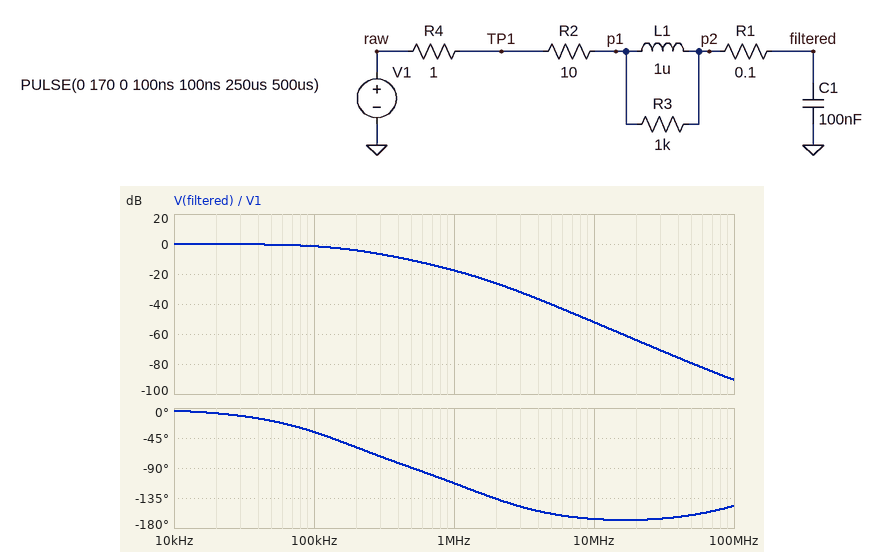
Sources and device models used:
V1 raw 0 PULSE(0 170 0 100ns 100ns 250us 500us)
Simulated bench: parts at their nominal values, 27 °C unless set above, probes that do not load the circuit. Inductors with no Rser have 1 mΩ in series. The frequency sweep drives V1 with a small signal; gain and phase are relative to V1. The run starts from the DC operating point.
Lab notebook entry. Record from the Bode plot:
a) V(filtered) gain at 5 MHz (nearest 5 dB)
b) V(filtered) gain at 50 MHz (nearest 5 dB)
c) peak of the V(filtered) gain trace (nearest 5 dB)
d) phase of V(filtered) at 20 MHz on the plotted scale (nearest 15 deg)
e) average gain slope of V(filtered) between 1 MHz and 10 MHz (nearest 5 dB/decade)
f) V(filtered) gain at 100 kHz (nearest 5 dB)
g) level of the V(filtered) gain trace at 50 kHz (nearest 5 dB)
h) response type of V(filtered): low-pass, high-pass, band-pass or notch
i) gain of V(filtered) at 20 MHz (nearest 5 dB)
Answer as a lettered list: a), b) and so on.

a) -40 dB
b) -80 dB
c) 0 dB
d) -165 deg
e) -35 dB/decade
f) 0 dB
g) 0 dB
h) low-pass
i) -65 dB
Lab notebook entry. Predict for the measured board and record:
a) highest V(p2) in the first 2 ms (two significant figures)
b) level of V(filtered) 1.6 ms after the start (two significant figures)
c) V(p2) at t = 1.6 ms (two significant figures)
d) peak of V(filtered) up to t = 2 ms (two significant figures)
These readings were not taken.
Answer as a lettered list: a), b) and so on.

a) 170 V
b) 170 V
c) 170 V
d) 170 V
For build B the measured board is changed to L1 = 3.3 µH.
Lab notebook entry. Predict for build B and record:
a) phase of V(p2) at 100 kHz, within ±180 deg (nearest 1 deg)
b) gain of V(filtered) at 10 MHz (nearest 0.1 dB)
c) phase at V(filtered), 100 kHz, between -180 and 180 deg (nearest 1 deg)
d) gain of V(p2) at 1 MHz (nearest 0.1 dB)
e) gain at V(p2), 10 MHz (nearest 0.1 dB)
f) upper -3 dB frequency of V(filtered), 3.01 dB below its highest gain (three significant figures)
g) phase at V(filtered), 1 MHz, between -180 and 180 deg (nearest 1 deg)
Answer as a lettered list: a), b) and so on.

a) -38 deg
b) -62.2 dB
c) -39 deg
d) -22.9 dB
e) -60.8 dB
f) 187 kHz
g) -149 deg
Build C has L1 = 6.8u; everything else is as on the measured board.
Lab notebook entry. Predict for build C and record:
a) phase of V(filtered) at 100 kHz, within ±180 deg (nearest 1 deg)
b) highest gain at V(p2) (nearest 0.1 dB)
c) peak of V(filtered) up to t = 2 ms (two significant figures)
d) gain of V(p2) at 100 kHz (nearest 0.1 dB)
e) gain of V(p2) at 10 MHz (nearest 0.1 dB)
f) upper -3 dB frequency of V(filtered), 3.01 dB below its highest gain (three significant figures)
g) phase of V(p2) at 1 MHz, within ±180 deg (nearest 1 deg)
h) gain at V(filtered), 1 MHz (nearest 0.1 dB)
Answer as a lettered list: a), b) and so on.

a) -44 deg
b) 0 dB
c) 180 V
d) -0.1 dB
e) -66.5 dB
f) 200 kHz
g) -159 deg
h) -28.6 dB
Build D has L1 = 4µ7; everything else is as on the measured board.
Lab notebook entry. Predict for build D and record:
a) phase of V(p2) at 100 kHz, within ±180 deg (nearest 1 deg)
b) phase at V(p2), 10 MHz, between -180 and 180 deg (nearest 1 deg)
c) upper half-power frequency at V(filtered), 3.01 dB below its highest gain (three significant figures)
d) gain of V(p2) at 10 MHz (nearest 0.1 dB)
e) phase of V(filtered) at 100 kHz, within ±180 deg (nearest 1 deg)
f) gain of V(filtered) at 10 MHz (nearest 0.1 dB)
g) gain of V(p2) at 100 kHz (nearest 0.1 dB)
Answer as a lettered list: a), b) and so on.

a) -40 deg
b) -129 deg
c) 198 kHz
d) -63.7 dB
e) -41 deg
f) -65.1 dB
g) -0.6 dB
